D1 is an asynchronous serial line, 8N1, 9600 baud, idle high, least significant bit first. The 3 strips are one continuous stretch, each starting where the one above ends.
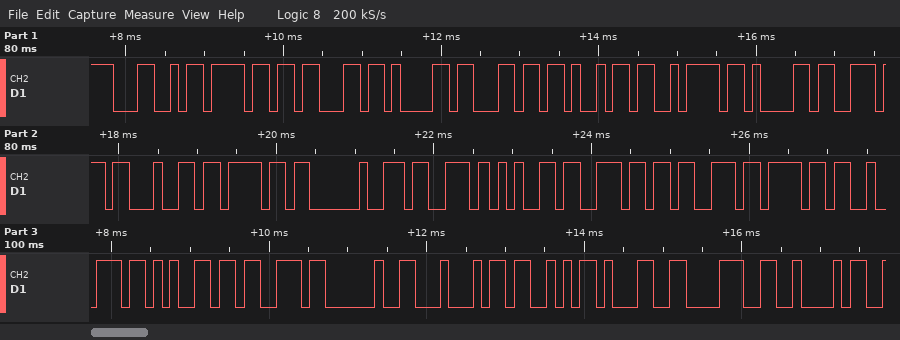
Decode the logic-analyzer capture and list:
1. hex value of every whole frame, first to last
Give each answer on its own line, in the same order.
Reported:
4C 6F 63 61 6C 69 7A 61 6E 64 6F 20 73 65 6E 73 6F 72 65 73 20 44 53 31 38 42
